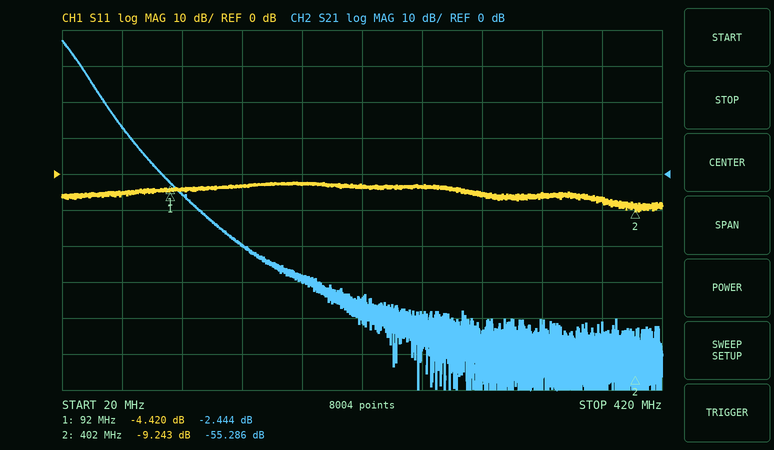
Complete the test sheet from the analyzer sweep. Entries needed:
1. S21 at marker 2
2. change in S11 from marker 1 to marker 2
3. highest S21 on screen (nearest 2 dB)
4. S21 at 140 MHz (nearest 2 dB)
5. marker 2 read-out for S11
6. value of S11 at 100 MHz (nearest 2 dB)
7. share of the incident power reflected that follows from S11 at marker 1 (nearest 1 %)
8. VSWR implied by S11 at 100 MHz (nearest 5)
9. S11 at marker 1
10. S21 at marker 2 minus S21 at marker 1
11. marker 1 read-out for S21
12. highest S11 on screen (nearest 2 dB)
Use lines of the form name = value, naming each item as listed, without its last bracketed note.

S21 at marker 2 = -55.286 dB
change in S11 from marker 1 to marker 2 = -4.823 dB
highest S21 on screen = 38 dB
S21 at 140 MHz = -20 dB
marker 2 read-out for S11 = -9.243 dB
value of S11 at 100 MHz = -4 dB
share of the incident power reflected that follows from S11 at marker 1 = 36 %
VSWR implied by S11 at 100 MHz = 5
S11 at marker 1 = -4.420 dB
S21 at marker 2 minus S21 at marker 1 = -52.842 dB
marker 1 read-out for S21 = -2.444 dB
highest S11 on screen = -2 dB
